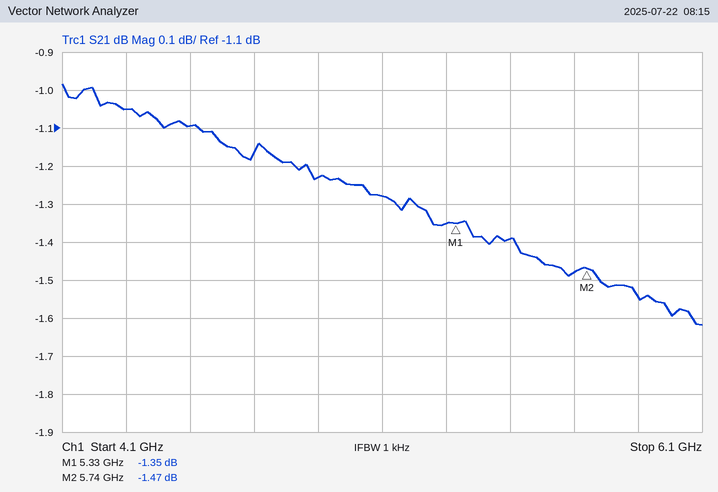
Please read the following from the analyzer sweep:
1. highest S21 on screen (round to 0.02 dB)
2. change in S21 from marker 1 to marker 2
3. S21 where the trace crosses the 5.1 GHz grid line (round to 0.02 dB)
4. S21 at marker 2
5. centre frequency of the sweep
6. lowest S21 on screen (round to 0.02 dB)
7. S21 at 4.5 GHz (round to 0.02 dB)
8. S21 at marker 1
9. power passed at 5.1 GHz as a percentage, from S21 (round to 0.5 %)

-0.98 dB
-0.12 dB
-1.28 dB
-1.47 dB
5.1 GHz
-1.62 dB
-1.10 dB
-1.35 dB
74.5 %
